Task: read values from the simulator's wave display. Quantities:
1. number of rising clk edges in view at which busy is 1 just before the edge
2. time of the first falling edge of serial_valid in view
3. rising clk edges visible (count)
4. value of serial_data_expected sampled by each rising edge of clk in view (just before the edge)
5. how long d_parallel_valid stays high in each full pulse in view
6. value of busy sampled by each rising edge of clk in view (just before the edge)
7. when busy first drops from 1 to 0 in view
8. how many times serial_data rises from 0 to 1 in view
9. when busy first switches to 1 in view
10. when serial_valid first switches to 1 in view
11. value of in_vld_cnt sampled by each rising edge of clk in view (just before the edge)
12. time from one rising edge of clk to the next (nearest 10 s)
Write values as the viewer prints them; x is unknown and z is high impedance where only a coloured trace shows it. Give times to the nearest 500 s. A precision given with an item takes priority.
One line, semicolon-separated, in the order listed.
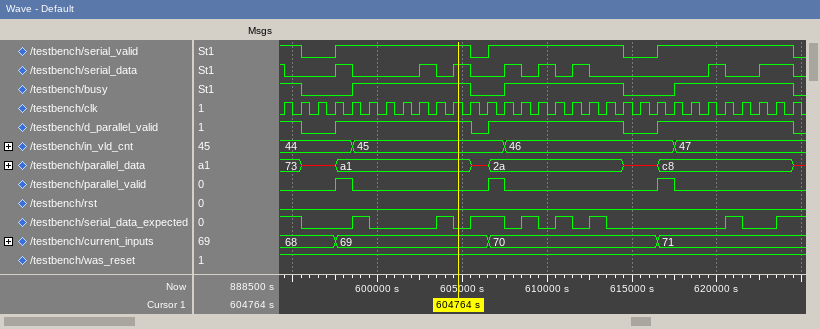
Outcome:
23; 595500 s; 31; 1 1 0 0 0 1 0 0 0 0 1 0 1 1 0 1 0 1 0 1 0 0 0 0 0 0 0 1 0 0 1; 8000 s, 8000 s, 8000 s; 1 1 0 0 0 1 1 1 1 1 1 1 0 0 1 1 1 1 1 1 1 0 0 0 1 1 1 1 1 1 1; 595500 s; 8; 598500 s; 597500 s; 44, 44, 44, 44, 44, 45, 45, 45, 45, 45, 45, 45, 45, 45, 46, 46, 46, 46, 46, 46, 46, 46, 46, 46, 47, 47, 47, 47, 47, 47, 47; 1000 s
